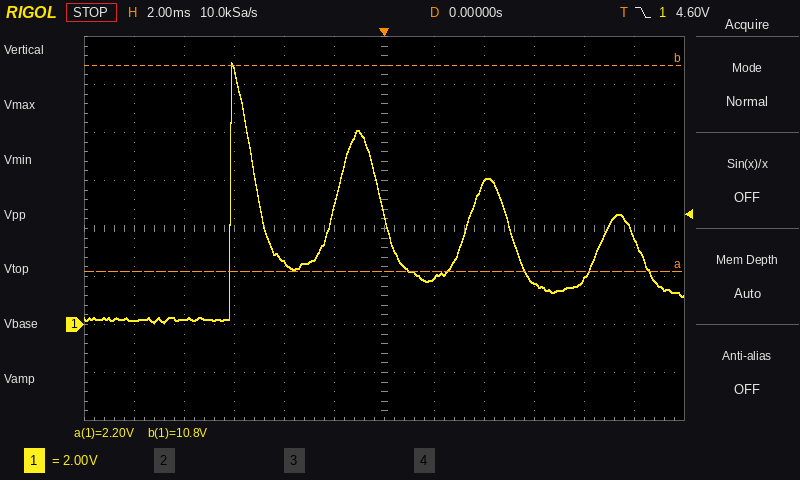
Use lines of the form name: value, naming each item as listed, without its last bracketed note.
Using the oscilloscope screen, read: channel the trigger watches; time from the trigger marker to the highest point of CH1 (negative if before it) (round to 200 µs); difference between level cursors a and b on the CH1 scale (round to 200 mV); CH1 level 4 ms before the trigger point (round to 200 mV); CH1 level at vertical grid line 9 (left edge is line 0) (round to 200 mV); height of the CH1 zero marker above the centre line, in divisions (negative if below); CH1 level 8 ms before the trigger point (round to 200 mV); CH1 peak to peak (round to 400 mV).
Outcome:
channel the trigger watches: CH1
time from the trigger marker to the highest point of CH1 (negative if before it): -6.0 ms
difference between level cursors a and b on the CH1 scale: 8.6 V
CH1 level 4 ms before the trigger point: 2.6 V
CH1 level at vertical grid line 9 (left edge is line 0): 1.8 V
height of the CH1 zero marker above the centre line, in divisions: -2.0 div
CH1 level 8 ms before the trigger point: 200 mV
CH1 peak to peak: 10.8 V
